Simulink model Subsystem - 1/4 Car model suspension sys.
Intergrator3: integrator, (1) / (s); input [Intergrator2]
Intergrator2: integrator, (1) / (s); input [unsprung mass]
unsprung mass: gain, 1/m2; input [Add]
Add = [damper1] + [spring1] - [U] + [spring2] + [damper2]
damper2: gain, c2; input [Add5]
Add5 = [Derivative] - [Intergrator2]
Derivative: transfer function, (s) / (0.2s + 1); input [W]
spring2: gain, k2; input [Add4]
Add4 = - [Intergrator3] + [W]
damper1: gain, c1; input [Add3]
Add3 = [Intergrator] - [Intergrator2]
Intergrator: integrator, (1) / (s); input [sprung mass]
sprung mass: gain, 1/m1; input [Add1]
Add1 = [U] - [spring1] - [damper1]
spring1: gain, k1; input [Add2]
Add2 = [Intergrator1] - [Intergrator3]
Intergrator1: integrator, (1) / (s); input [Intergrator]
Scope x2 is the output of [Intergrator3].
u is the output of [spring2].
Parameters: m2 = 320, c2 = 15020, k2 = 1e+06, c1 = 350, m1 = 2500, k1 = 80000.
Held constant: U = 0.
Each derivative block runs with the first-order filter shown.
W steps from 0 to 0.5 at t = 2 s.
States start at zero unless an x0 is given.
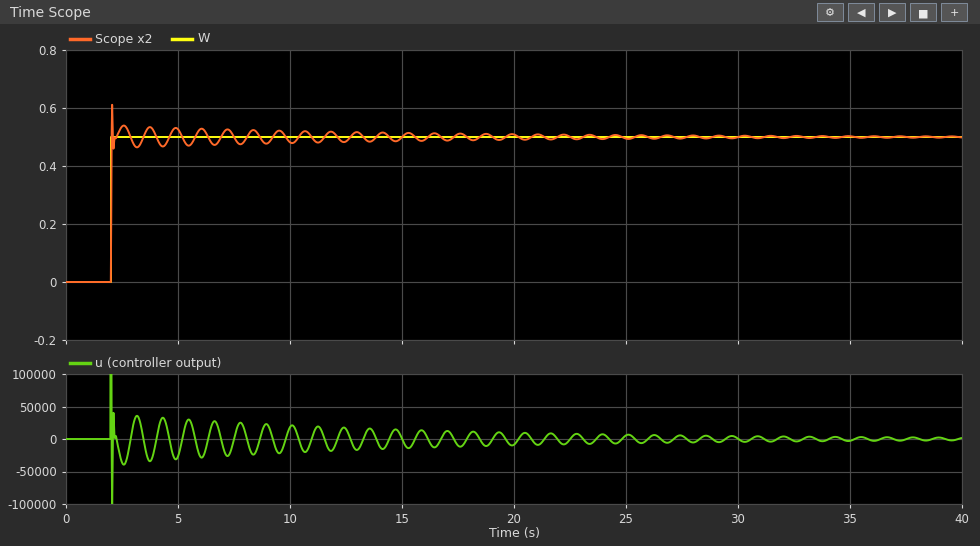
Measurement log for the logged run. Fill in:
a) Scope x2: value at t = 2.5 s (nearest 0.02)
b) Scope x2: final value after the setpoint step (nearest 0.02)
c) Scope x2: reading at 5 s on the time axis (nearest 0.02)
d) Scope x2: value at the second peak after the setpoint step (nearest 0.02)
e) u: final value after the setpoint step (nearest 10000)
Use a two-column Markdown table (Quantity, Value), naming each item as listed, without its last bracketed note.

| Quantity | Value |
|---|---|
| Scope x2: value at t = 2.5 s | 0.54 |
| Scope x2: final value after the setpoint step | 0.50 |
| Scope x2: reading at 5 s on the time axis | 0.52 |
| Scope x2: value at the second peak after the setpoint step | 0.54 |
| u: final value after the setpoint step | 0 |
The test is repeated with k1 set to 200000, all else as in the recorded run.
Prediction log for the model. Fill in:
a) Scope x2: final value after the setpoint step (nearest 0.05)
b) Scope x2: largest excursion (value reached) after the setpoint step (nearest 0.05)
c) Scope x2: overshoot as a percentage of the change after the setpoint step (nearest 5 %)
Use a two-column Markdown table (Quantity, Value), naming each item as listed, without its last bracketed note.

| Quantity | Value |
|---|---|
| Scope x2: final value after the setpoint step | 0.50 |
| Scope x2: largest excursion (value reached) after the setpoint step | 0.60 |
| Scope x2: overshoot as a percentage of the change after the setpoint step | 20 % |
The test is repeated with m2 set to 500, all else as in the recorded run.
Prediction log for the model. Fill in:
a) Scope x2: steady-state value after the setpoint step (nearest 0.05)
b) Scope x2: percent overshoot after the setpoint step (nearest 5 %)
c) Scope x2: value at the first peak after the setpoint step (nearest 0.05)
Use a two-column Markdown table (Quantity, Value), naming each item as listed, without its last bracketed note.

| Quantity | Value |
|---|---|
| Scope x2: steady-state value after the setpoint step | 0.50 |
| Scope x2: percent overshoot after the setpoint step | 30 % |
| Scope x2: value at the first peak after the setpoint step | 0.65 |
